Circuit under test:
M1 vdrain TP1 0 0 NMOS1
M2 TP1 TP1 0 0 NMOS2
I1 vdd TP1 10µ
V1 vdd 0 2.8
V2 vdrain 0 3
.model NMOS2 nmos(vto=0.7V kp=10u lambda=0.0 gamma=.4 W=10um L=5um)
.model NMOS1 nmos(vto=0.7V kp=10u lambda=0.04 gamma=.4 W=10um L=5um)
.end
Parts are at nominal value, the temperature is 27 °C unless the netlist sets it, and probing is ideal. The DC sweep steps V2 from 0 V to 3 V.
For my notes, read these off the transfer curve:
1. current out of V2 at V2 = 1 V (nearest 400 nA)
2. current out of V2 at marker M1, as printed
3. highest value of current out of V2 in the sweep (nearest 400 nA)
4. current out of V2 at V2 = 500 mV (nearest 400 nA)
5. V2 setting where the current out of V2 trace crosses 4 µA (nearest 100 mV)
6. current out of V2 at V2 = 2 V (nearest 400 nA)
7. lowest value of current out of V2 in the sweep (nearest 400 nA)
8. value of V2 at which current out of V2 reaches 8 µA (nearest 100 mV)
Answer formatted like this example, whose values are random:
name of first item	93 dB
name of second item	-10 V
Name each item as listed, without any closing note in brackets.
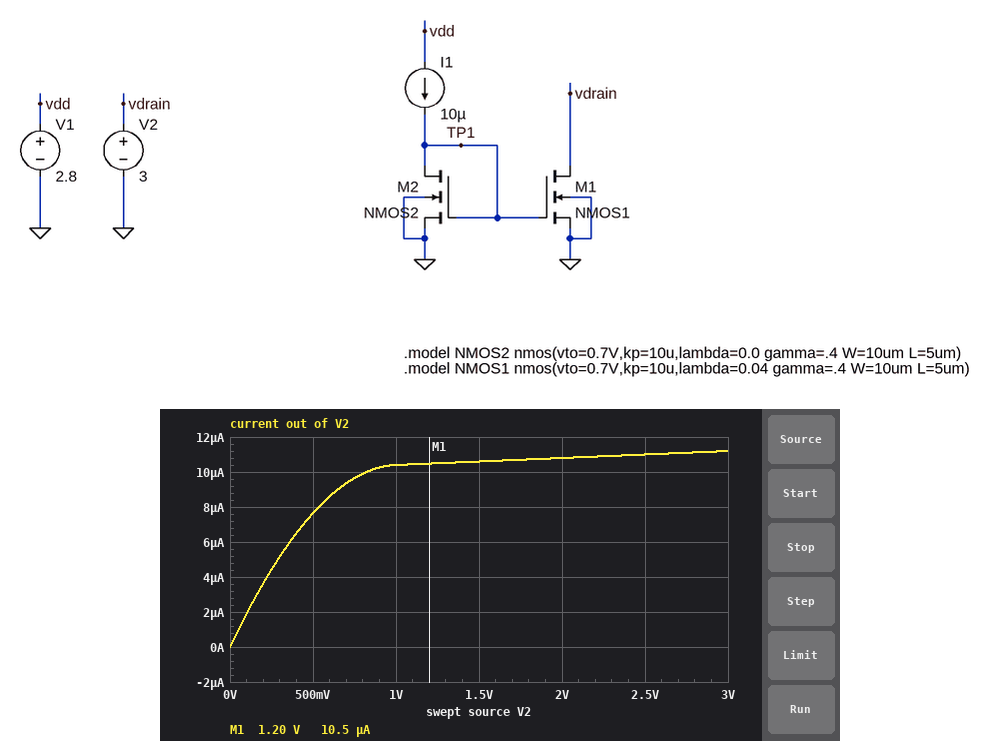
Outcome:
current out of V2 at V2 = 1 V	10.4 µA
current out of V2 at marker M1, as printed	10.5 µA
highest value of current out of V2 in the sweep	11.2 µA
current out of V2 at V2 = 500 mV	7.6 µA
V2 setting where the current out of V2 trace crosses 4 µA	200 mV
current out of V2 at V2 = 2 V	10.8 µA
lowest value of current out of V2 in the sweep	0 A
value of V2 at which current out of V2 reaches 8 µA	500 mV
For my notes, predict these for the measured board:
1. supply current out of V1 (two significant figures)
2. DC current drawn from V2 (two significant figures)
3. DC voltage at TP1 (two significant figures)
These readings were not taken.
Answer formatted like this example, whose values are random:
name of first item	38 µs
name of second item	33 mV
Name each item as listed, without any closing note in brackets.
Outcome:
supply current out of V1	10 µA
DC current drawn from V2	11 µA
DC voltage at TP1	1.7 V
